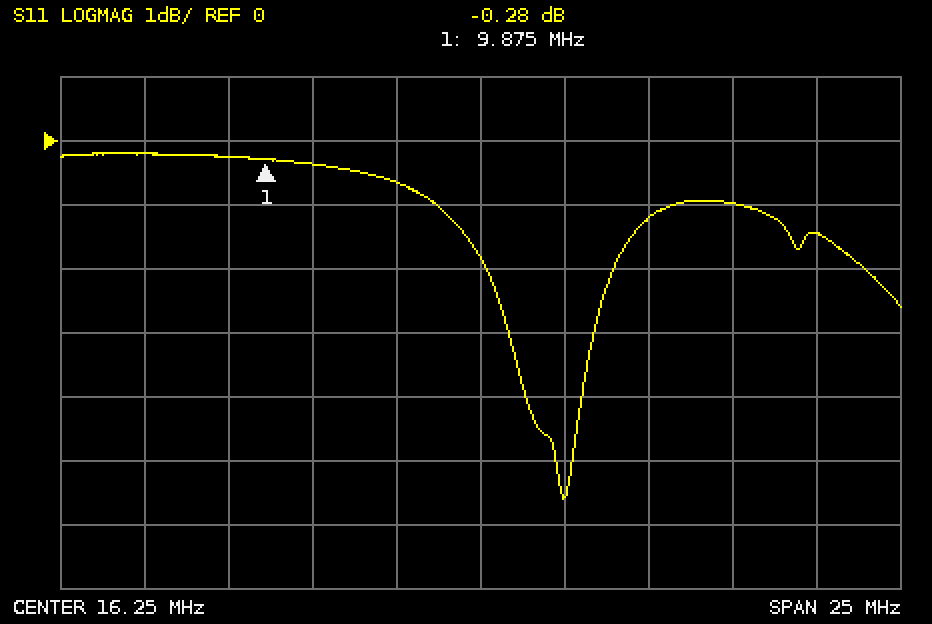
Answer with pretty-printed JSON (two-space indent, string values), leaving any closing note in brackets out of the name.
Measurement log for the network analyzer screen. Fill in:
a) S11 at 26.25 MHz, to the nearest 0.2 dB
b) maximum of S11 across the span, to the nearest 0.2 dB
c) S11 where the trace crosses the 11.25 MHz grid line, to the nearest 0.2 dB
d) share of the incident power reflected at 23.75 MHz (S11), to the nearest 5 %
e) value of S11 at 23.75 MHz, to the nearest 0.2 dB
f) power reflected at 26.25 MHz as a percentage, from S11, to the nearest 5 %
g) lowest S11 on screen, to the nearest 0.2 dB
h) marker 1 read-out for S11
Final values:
{
  "S11 at 26.25 MHz, to the nearest 0.2 dB": "-1.4 dB",
  "maximum of S11 across the span, to the nearest 0.2 dB": "-0.2 dB",
  "S11 where the trace crosses the 11.25 MHz grid line, to the nearest 0.2 dB": "-0.4 dB",
  "share of the incident power reflected at 23.75 MHz (S11), to the nearest 5 %": "80 %",
  "value of S11 at 23.75 MHz, to the nearest 0.2 dB": "-1.0 dB",
  "power reflected at 26.25 MHz as a percentage, from S11, to the nearest 5 %": "70 %",
  "lowest S11 on screen, to the nearest 0.2 dB": "-5.6 dB",
  "marker 1 read-out for S11": "-0.28 dB"
}
